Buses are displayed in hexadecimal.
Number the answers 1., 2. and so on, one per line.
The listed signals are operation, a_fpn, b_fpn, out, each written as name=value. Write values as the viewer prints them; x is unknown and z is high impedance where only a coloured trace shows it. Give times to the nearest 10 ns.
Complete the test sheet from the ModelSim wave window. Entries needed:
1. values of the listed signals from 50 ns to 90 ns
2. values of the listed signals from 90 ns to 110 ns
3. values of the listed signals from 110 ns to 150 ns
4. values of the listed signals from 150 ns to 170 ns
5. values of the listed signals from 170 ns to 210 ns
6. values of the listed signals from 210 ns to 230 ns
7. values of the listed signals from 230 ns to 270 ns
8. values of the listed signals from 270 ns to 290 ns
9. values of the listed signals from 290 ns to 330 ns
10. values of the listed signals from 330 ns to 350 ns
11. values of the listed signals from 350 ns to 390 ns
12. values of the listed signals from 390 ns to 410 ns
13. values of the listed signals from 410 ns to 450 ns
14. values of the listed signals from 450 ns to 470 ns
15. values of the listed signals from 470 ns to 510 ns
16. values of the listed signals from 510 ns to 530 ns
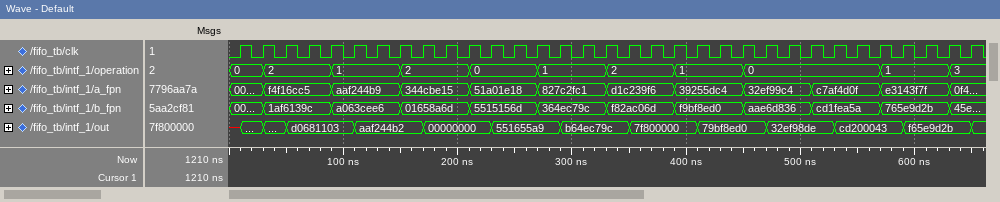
1. operation=2, a_fpn=f4f16cc5, b_fpn=1af6139c, out=d0681103
2. operation=1, a_fpn=aaf244b9, b_fpn=a063cee6, out=d0681103
3. operation=1, a_fpn=aaf244b9, b_fpn=a063cee6, out=aaf244b2
4. operation=2, a_fpn=344cbe15, b_fpn=01658a6d, out=aaf244b2
5. operation=2, a_fpn=344cbe15, b_fpn=01658a6d, out=00000000
6. operation=0, a_fpn=51a01e18, b_fpn=5515156d, out=00000000
7. operation=0, a_fpn=51a01e18, b_fpn=5515156d, out=551655a9
8. operation=1, a_fpn=827c2fc1, b_fpn=364ec79c, out=551655a9
9. operation=1, a_fpn=827c2fc1, b_fpn=364ec79c, out=b64ec79c
10. operation=2, a_fpn=d1c239f6, b_fpn=f82ac06d, out=b64ec79c
11. operation=2, a_fpn=d1c239f6, b_fpn=f82ac06d, out=7f800000
12. operation=1, a_fpn=39255dc4, b_fpn=f9bf8ed0, out=7f800000
13. operation=1, a_fpn=39255dc4, b_fpn=f9bf8ed0, out=79bf8ed0
14. operation=0, a_fpn=32ef99c4, b_fpn=aae6d836, out=79bf8ed0
15. operation=0, a_fpn=32ef99c4, b_fpn=aae6d836, out=32ef98de
16. operation=0, a_fpn=c7af4d0f, b_fpn=cd1fea5a, out=32ef98de
